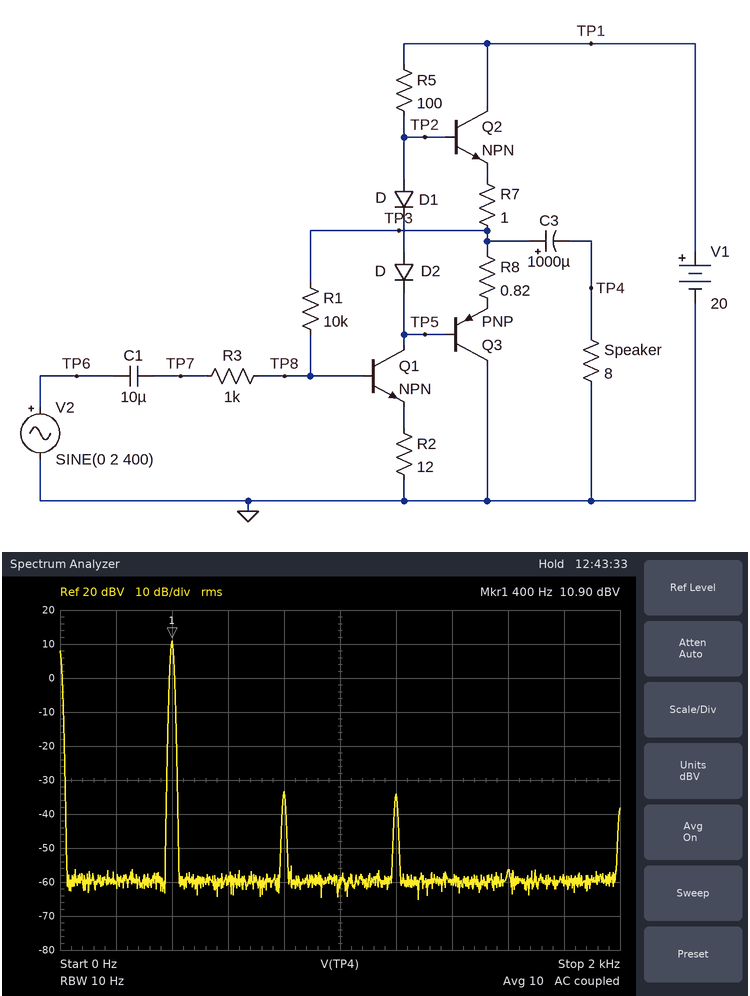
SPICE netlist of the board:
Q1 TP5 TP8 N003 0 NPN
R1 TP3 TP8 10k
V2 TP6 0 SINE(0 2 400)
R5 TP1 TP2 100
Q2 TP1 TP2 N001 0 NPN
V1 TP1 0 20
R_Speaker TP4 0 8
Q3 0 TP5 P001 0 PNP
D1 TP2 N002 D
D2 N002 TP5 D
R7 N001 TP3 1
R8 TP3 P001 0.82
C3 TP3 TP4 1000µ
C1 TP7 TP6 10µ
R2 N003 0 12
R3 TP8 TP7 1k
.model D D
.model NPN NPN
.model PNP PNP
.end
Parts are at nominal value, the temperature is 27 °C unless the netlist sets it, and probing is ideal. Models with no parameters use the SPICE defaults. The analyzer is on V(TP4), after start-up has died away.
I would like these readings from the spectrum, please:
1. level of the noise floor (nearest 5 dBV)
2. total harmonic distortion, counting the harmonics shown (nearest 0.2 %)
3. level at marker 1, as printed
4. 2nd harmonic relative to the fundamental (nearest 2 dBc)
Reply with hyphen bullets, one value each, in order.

- -60 dBV
- 0.8 %
- 10.90 dBV
- -44 dBc
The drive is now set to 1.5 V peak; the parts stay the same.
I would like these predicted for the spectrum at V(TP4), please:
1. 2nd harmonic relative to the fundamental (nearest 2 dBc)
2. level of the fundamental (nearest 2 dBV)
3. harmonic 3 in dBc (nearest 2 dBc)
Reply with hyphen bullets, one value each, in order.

- -46 dBc
- 8 dBV
- -42 dBc
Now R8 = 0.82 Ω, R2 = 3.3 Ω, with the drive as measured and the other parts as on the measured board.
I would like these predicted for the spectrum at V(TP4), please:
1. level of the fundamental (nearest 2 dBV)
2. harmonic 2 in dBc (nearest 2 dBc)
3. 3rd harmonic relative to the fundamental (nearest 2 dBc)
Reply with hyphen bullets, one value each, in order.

- 14 dBV
- -38 dBc
- -56 dBc
